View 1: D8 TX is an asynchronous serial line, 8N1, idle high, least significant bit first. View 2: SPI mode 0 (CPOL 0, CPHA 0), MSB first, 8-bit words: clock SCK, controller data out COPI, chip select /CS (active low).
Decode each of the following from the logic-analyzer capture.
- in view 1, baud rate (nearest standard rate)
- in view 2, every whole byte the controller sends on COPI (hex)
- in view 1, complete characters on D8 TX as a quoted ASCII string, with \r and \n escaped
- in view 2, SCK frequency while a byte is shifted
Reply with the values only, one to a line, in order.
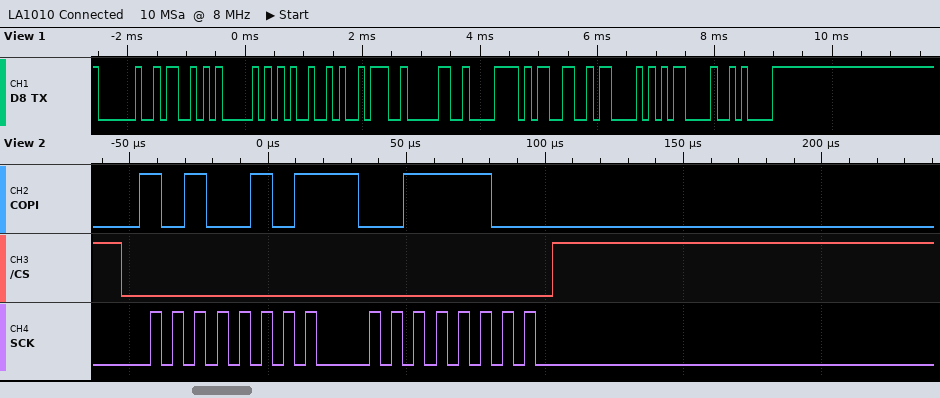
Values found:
9600 baud
A5 3C
" SPI:0x3C\r\n"
125 kHz
